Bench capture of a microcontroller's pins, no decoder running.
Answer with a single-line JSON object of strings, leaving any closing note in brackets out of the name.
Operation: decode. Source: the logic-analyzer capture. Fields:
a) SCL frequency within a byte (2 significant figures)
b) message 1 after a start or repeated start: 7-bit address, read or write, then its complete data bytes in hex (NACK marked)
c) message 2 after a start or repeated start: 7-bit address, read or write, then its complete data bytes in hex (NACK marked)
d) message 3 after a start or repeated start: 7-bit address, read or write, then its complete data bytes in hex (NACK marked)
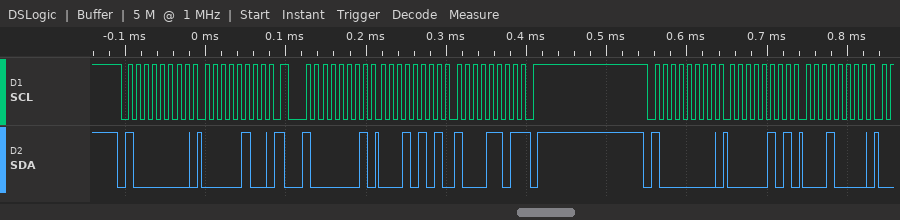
{"SCL frequency within a byte": "100 kHz", "message 1 after a start or repeated start: 7-bit address, read or write, then its complete data bytes in hex": "0x40 write: 04", "message 2 after a start or repeated start: 7-bit address, read or write, then its complete data bytes in hex": "0x40 read: 15 8D NACK", "message 3 after a start or repeated start: 7-bit address, read or write, then its complete data bytes in hex": "0x40 write: 05 10"}
